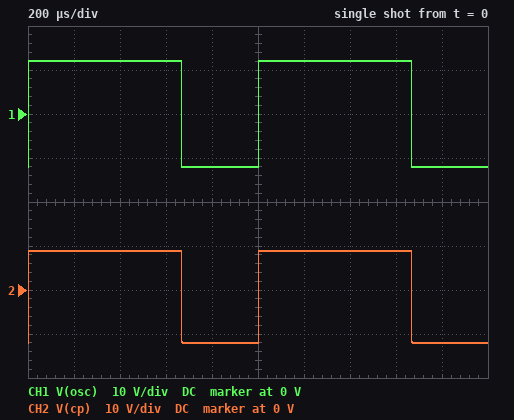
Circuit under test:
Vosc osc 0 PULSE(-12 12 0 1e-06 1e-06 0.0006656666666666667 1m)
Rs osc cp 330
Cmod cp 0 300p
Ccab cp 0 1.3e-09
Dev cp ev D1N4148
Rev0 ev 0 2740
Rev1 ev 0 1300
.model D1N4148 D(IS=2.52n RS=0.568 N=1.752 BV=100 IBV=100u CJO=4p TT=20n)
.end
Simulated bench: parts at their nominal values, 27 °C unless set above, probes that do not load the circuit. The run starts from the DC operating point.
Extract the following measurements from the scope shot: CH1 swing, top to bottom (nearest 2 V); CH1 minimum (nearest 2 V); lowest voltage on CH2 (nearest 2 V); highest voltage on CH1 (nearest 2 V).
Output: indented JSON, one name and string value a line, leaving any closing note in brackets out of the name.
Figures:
{
  "CH1 swing, top to bottom": "24 V",
  "CH1 minimum": "-12 V",
  "lowest voltage on CH2": "-12 V",
  "highest voltage on CH1": "12 V"
}
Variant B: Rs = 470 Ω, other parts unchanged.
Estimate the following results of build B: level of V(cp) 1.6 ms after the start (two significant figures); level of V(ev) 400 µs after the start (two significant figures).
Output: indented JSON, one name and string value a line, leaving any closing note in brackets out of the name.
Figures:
{
  "level of V(cp) 1.6 ms after the start": "8.1 V",
  "level of V(ev) 400 µs after the start": "7.4 V"
}
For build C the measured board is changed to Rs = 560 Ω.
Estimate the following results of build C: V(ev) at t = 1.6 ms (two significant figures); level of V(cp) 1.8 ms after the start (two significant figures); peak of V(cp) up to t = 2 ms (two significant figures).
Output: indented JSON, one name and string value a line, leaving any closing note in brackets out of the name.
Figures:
{
  "V(ev) at t = 1.6 ms": "6.9 V",
  "level of V(cp) 1.8 ms after the start": "-12 V",
  "peak of V(cp) up to t = 2 ms": "7.6 V"
}
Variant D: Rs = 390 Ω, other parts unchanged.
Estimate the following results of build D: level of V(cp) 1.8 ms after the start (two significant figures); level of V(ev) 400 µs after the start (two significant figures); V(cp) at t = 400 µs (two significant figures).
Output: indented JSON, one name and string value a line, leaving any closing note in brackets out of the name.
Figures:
{
  "level of V(cp) 1.8 ms after the start": "-12 V",
  "level of V(ev) 400 µs after the start": "7.8 V",
  "V(cp) at t = 400 µs": "8.5 V"
}
